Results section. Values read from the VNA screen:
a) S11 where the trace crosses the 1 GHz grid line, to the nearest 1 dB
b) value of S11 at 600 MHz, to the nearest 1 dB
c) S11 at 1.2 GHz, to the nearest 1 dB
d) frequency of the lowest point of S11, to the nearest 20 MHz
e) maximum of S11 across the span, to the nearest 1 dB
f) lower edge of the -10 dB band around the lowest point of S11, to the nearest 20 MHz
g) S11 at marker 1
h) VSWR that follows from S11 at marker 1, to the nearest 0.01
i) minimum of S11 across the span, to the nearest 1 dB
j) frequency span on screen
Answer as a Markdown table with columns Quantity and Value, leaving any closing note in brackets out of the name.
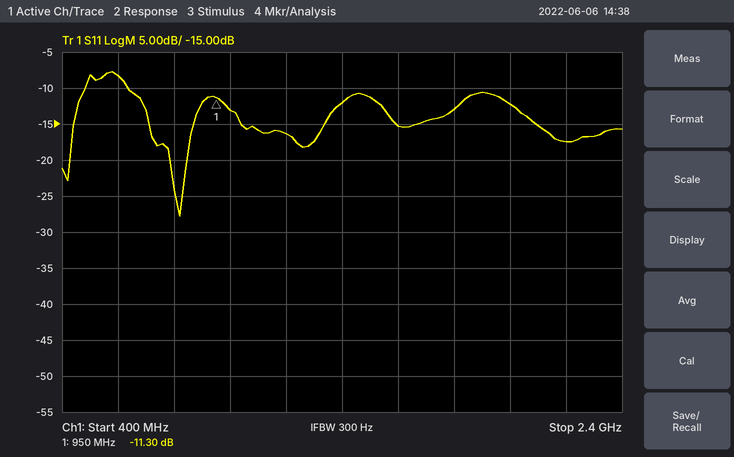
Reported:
| Quantity | Value |
|---|---|
| S11 where the trace crosses the 1 GHz grid line, to the nearest 1 dB | -13 dB |
| value of S11 at 600 MHz, to the nearest 1 dB | -8 dB |
| S11 at 1.2 GHz, to the nearest 1 dB | -16 dB |
| frequency of the lowest point of S11, to the nearest 20 MHz | 820 MHz |
| maximum of S11 across the span, to the nearest 1 dB | -8 dB |
| lower edge of the -10 dB band around the lowest point of S11, to the nearest 20 MHz | 640 MHz |
| S11 at marker 1 | -11.30 dB |
| VSWR that follows from S11 at marker 1, to the nearest 0.01 | 1.75 |
| minimum of S11 across the span, to the nearest 1 dB | -28 dB |
| frequency span on screen | 2 GHz |
